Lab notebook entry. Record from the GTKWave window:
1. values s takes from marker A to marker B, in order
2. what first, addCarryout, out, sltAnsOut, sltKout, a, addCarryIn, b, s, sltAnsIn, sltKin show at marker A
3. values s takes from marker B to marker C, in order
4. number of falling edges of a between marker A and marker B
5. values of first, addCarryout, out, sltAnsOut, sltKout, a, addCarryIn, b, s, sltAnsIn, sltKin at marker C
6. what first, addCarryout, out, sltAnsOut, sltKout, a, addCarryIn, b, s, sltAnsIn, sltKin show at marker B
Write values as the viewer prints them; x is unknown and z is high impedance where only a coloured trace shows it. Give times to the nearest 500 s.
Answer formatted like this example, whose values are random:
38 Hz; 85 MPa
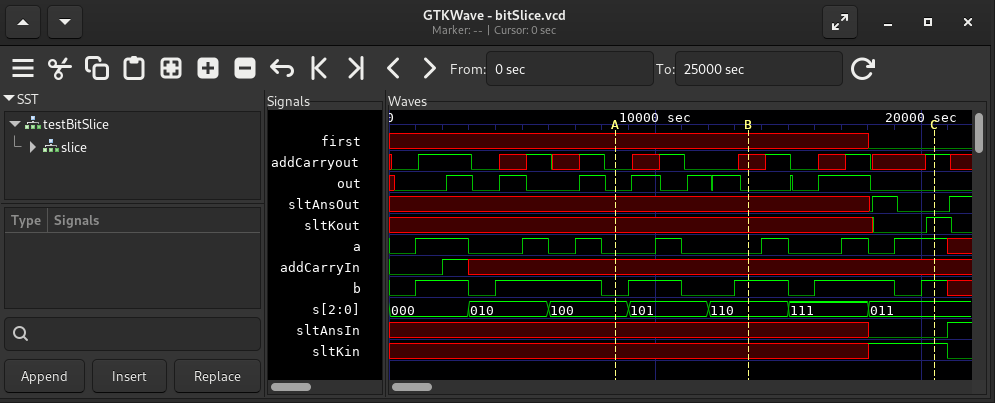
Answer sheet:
100, 101, 110; first=x, addCarryout=0, out=0, sltAnsOut=x, sltKout=x, a=0, addCarryIn=x, b=0, s=100, sltAnsIn=x, sltKin=x; 110, 111, 011; 1; first=0, addCarryout=1, out=0, sltAnsOut=0, sltKout=1, a=1, addCarryIn=x, b=1, s=011, sltAnsIn=0, sltKin=1; first=x, addCarryout=x, out=0, sltAnsOut=x, sltKout=x, a=0, addCarryIn=x, b=1, s=110, sltAnsIn=x, sltKin=x
